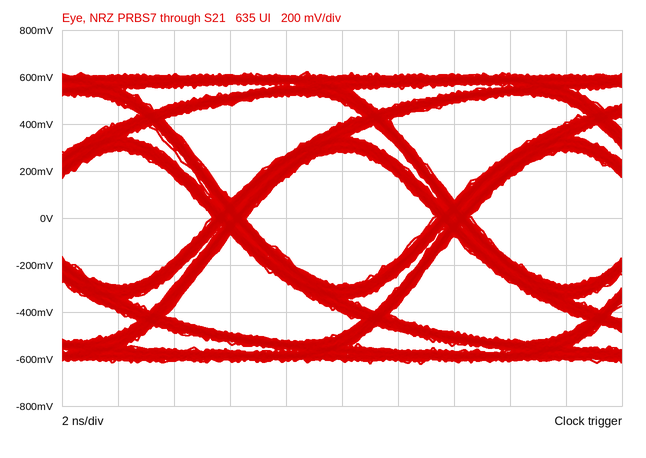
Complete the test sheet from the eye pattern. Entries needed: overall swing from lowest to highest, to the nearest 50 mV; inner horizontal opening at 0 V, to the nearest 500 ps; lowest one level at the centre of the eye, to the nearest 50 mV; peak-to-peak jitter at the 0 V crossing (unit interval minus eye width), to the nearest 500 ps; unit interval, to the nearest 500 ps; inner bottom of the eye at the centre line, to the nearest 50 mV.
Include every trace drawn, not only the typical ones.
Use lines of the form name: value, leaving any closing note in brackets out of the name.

overall swing from lowest to highest, to the nearest 50 mV: 1.25 V
inner horizontal opening at 0 V, to the nearest 500 ps: 6.5 ns
lowest one level at the centre of the eye, to the nearest 50 mV: 300 mV
peak-to-peak jitter at the 0 V crossing (unit interval minus eye width), to the nearest 500 ps: 1.5 ns
unit interval, to the nearest 500 ps: 8.0 ns
inner bottom of the eye at the centre line, to the nearest 50 mV: -300 mV
